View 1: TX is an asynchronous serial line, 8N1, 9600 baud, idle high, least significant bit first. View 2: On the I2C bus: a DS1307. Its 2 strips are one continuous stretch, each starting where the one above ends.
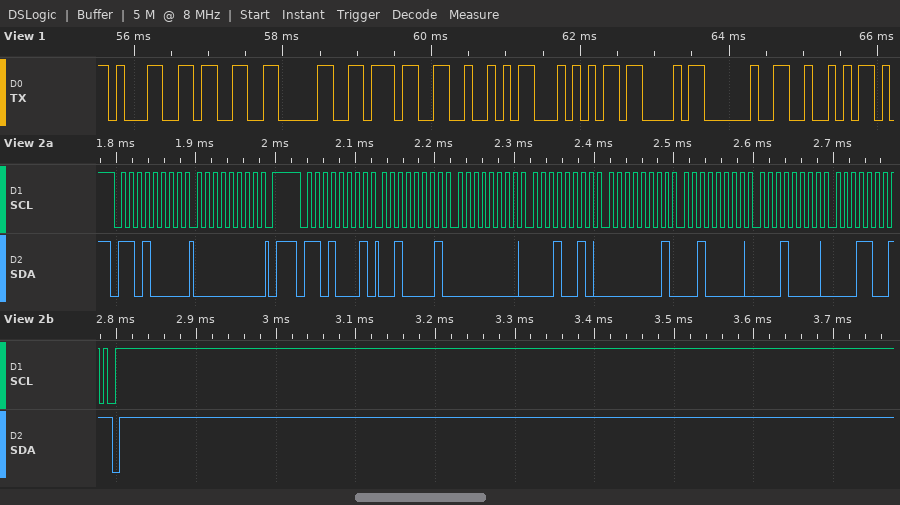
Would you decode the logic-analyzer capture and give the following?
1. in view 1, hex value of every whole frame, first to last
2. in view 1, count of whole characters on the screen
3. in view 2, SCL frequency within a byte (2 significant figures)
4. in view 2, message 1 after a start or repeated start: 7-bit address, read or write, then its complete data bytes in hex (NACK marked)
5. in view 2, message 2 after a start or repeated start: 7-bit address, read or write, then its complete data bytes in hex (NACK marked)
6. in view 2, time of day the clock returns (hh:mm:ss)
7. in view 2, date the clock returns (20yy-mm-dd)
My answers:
31 33 30 37 52 54 43 20 52
9
100 kHz
0x68 write: 00
0x68 read: 21 00 12 01 20 10 19 NACK
12:00:21
2019-10-20
